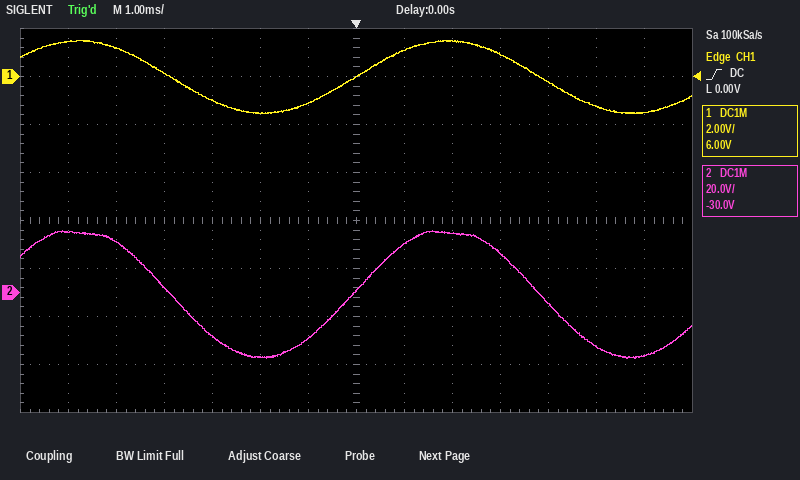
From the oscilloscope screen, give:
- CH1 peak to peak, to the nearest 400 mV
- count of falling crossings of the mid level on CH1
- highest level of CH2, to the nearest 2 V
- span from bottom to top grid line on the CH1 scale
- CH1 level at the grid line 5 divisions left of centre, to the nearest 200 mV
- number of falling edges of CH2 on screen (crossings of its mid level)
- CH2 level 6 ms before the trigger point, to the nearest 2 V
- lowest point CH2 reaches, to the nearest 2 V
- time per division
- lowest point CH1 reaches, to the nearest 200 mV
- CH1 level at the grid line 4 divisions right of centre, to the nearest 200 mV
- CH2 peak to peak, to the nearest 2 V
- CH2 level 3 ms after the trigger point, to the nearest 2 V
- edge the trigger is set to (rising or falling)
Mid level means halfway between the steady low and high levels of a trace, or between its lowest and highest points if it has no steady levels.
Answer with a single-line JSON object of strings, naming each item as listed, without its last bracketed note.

{"CH1 peak to peak, to the nearest 400 mV": "3.2 V", "count of falling crossings of the mid level on CH1": "2", "highest level of CH2, to the nearest 2 V": "26 V", "span from bottom to top grid line on the CH1 scale": "16 V", "CH1 level at the grid line 5 divisions left of centre, to the nearest 200 mV": "1.2 V", "number of falling edges of CH2 on screen": "2", "CH2 level 6 ms before the trigger point, to the nearest 2 V": "26 V", "lowest point CH2 reaches, to the nearest 2 V": "-28 V", "time per division": "1 ms", "lowest point CH1 reaches, to the nearest 200 mV": "-1.6 V", "CH1 level at the grid line 4 divisions right of centre, to the nearest 200 mV": "-200 mV", "CH2 peak to peak, to the nearest 2 V": "54 V", "CH2 level 3 ms after the trigger point, to the nearest 2 V": "16 V", "edge the trigger is set to": "rising"}
